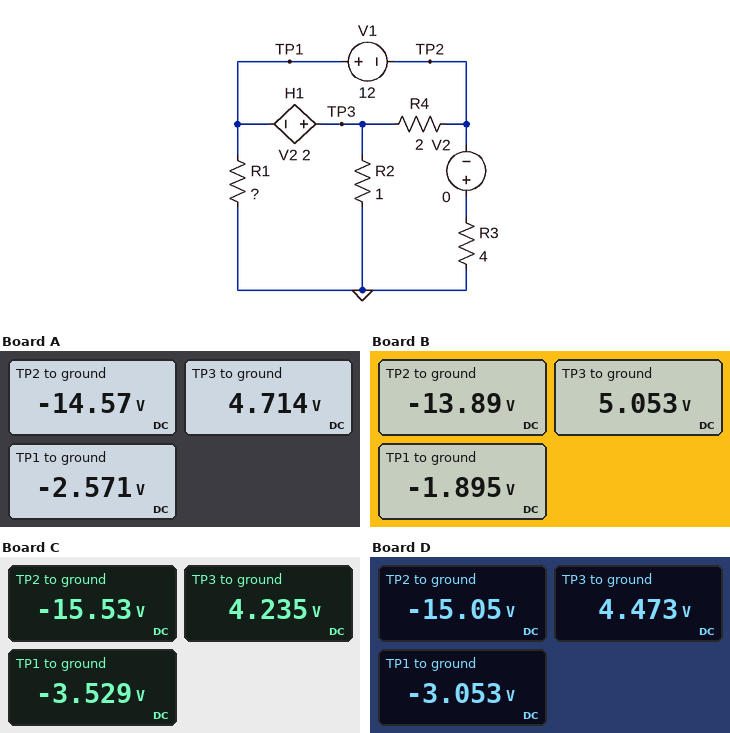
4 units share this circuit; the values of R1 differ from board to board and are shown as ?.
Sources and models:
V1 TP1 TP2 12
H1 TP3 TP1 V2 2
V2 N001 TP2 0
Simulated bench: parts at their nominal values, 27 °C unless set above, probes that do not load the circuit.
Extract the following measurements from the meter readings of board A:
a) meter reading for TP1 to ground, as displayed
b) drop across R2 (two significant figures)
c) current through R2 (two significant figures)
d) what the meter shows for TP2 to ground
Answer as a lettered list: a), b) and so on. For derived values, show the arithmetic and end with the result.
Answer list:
a) -2.571 V
b) 4.714 V = 4.7 V
c) (4.714 V) / 1 Ω = 4.7 A
d) -14.57 V
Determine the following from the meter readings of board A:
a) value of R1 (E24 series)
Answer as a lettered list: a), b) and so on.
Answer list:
a) 2.4 Ω
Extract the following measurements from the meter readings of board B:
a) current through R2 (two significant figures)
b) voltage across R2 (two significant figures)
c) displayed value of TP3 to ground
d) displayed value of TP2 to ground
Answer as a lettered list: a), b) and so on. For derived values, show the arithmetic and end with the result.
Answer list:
a) (5.053 V) / 1 Ω = 5.1 A
b) 5.053 V = 5.1 V
c) 5.053 V
d) -13.89 V
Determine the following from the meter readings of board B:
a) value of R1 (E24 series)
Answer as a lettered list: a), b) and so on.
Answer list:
a) 1.2 Ω
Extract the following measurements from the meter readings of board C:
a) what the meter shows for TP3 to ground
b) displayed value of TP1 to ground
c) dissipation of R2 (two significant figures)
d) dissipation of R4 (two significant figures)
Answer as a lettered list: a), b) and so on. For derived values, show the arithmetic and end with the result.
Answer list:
a) 4.235 V
b) -3.529 V
c) (4.235 V)^2 / 1 Ω = 18 W
d) (4.235 V - (-15.53 V))^2 / 2 Ω = 200 W
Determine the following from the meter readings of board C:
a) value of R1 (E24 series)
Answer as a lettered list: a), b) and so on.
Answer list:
a) 10 Ω
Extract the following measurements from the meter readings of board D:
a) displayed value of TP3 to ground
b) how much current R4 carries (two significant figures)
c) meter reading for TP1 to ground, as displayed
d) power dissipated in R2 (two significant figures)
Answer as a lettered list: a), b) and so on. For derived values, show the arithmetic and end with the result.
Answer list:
a) 4.473 V
b) (4.473 V - (-15.05 V)) / 2 Ω = 9.8 A
c) -3.053 V
d) (4.473 V)^2 / 1 Ω = 20 W
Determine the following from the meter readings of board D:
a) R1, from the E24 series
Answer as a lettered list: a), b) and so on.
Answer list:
a) 4.3 Ω
